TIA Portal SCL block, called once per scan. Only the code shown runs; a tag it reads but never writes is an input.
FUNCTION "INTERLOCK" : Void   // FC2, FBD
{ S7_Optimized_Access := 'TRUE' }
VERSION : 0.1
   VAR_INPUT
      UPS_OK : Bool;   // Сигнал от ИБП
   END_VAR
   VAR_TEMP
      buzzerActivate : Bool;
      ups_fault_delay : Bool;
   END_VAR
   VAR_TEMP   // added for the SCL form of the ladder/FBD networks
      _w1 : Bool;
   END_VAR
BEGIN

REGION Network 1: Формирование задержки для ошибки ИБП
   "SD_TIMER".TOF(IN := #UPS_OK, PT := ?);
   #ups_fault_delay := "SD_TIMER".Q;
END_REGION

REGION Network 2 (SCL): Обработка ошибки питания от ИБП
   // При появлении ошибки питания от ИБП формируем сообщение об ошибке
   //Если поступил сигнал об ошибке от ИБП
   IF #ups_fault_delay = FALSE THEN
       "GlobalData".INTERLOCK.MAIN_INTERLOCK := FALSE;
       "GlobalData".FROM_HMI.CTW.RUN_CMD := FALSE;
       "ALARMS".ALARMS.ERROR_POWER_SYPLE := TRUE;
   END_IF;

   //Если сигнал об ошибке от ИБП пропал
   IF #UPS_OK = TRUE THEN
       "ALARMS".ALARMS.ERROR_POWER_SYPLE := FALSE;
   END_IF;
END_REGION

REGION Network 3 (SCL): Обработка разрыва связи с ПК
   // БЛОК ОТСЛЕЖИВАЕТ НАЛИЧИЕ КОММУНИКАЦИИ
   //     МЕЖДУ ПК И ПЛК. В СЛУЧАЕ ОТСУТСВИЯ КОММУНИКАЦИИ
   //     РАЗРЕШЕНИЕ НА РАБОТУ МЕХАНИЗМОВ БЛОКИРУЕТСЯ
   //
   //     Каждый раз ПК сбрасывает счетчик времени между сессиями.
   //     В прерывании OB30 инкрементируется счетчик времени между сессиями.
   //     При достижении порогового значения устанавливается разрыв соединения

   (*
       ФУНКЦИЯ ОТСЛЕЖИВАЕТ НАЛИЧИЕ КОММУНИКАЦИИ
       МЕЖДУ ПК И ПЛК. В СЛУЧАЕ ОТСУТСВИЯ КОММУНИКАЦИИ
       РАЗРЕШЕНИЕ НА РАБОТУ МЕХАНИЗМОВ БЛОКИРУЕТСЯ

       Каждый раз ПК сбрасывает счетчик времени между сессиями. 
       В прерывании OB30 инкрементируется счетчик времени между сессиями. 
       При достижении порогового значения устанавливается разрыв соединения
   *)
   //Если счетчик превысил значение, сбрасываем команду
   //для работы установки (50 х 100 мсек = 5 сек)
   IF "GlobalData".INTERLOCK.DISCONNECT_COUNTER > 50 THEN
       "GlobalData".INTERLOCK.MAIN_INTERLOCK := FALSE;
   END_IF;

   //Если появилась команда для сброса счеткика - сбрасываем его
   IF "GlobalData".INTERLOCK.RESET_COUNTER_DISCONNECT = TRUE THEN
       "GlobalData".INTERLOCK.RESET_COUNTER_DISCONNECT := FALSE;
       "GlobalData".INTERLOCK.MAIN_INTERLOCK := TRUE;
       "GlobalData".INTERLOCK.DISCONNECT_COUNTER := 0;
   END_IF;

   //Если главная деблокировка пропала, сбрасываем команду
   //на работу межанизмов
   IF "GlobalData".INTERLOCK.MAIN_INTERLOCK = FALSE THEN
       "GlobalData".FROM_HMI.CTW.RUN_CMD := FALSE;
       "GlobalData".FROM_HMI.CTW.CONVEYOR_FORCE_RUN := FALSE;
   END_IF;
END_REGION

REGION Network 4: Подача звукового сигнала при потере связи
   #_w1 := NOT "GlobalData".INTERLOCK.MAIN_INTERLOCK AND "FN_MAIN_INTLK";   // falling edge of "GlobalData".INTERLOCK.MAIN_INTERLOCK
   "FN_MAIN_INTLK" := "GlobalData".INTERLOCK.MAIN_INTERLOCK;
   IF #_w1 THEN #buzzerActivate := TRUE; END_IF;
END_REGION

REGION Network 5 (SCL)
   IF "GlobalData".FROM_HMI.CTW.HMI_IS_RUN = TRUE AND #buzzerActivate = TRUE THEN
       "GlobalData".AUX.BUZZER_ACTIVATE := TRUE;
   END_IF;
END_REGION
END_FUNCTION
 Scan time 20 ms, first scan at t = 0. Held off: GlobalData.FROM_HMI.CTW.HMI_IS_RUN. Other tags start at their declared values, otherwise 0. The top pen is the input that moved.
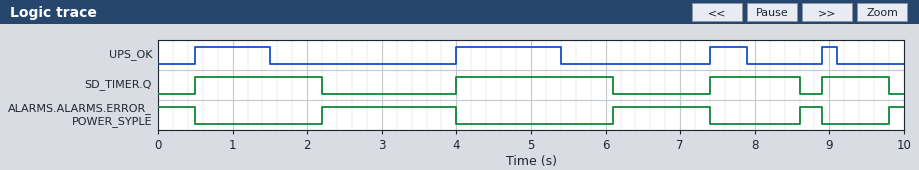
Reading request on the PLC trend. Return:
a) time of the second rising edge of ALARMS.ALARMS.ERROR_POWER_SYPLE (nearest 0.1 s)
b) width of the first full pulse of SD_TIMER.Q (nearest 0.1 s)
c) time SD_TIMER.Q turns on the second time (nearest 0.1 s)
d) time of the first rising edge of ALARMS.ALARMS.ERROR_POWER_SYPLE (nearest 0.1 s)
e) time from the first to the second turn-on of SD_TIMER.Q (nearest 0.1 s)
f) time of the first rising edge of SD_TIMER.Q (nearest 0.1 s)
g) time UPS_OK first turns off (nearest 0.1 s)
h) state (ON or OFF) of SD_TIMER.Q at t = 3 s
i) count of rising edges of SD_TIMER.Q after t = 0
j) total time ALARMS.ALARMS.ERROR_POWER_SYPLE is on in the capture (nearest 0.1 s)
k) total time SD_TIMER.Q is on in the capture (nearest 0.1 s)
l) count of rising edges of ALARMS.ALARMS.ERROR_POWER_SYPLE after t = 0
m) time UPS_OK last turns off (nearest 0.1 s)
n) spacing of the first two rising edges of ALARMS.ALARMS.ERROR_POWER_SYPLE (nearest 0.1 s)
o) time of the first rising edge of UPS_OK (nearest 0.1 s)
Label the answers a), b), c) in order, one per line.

a) 6.1 s
b) 1.7 s
c) 4.0 s
d) 2.2 s
e) 3.5 s
f) 0.5 s
g) 1.5 s
h) OFF
i) 4
j) 4.1 s
k) 5.9 s
l) 4
m) 9.1 s
n) 3.9 s
o) 0.5 s
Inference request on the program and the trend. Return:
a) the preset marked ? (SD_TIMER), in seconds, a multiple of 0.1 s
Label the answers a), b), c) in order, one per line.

a) 0.7 s
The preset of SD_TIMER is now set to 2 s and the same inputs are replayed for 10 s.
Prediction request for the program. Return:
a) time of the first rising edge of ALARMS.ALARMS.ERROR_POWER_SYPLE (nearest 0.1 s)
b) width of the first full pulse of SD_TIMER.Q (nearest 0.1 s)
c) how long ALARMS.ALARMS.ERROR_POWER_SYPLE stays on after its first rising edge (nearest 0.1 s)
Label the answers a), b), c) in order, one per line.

a) 3.5 s
b) 3.0 s
c) 0.5 s
